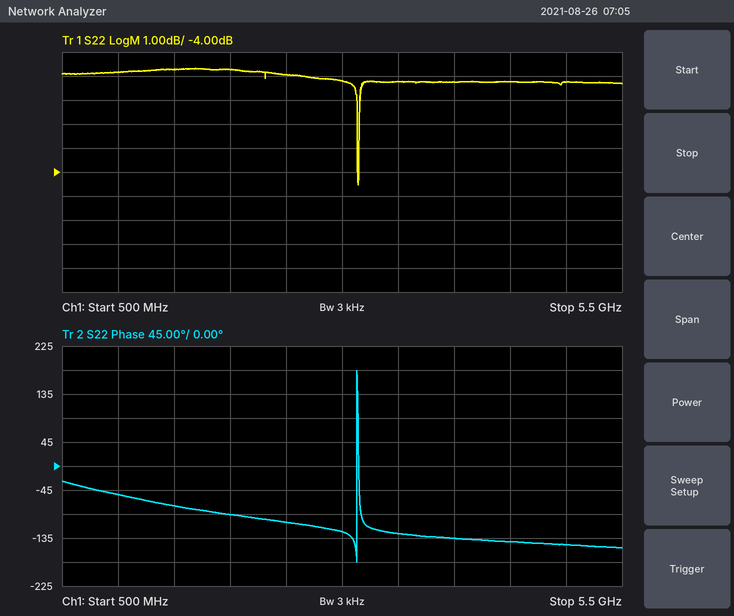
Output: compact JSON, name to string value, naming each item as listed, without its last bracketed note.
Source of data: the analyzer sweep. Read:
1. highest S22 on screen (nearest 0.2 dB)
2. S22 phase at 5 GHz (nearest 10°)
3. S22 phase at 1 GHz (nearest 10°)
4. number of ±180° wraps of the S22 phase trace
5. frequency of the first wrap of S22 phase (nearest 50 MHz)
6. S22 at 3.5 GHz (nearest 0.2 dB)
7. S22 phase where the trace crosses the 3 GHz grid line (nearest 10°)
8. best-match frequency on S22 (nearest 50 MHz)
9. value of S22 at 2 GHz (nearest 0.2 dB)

{"highest S22 on screen": "0.4 dB", "S22 phase at 5 GHz": "-150°", "S22 phase at 1 GHz": "-50°", "number of ±180° wraps of the S22 phase trace": "1", "frequency of the first wrap of S22 phase": "3.15 GHz", "S22 at 3.5 GHz": "-0.2 dB", "S22 phase where the trace crosses the 3 GHz grid line": "-120°", "best-match frequency on S22": "3.15 GHz", "value of S22 at 2 GHz": "0.2 dB"}
